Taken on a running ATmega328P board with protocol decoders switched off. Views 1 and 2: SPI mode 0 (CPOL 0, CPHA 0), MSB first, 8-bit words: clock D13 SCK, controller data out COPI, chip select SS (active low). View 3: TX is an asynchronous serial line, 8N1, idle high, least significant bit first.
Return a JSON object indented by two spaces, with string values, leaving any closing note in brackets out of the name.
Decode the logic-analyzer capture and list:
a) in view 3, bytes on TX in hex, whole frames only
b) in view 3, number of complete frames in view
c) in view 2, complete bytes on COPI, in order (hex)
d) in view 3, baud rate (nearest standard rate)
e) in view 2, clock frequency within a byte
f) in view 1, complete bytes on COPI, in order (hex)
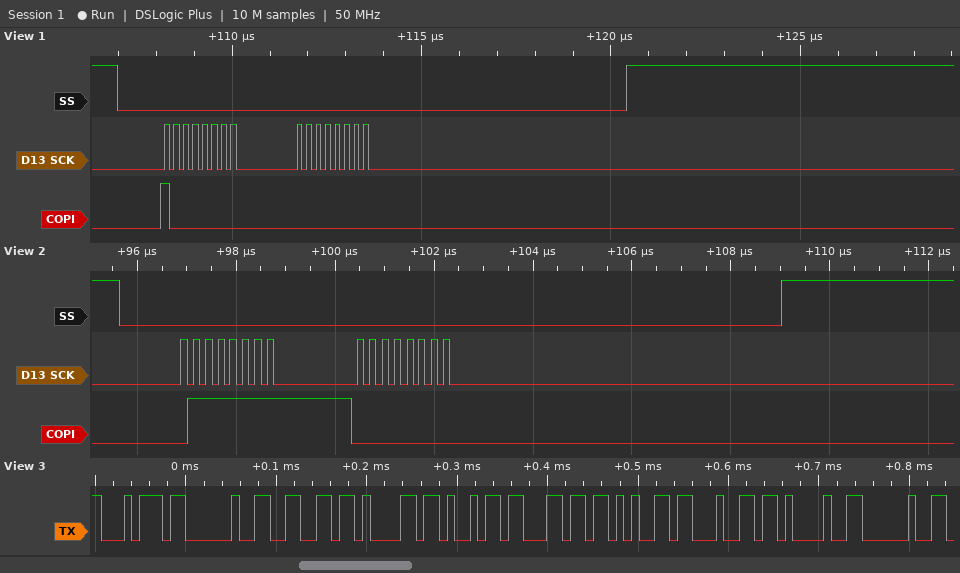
{
  "in view 3, bytes on TX in hex, whole frames only": "0x74 0x20 0x66 0x61 0x69 0x6C 0x65 0x64 0x21 0x20",
  "in view 3, number of complete frames in view": "10",
  "in view 2, complete bytes on COPI, in order": "7F 00",
  "in view 3, baud rate": "115200 baud",
  "in view 2, clock frequency within a byte": "4 MHz",
  "in view 1, complete bytes on COPI, in order": "80 00"
}
